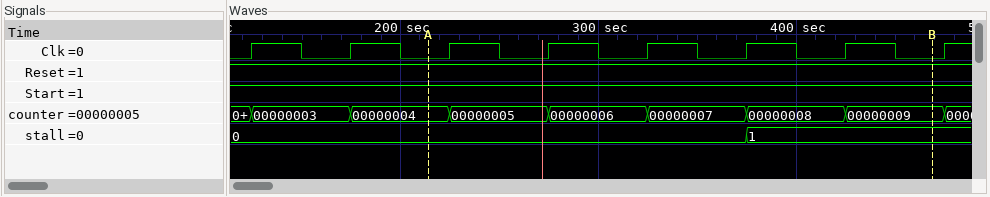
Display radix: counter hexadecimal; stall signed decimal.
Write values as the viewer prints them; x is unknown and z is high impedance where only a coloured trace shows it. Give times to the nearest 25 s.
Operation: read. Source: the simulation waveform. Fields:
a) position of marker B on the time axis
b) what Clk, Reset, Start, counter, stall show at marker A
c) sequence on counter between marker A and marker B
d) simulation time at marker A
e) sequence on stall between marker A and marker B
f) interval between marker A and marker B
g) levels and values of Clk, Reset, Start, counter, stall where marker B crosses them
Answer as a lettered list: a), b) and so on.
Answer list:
a) 475 s
b) Clk=0, Reset=1, Start=1, counter=00000004, stall=0
c) 00000004, 00000005, 00000006, 00000007, 00000008, 00000009
d) 225 s
e) 0, 1
f) 250 s
g) Clk=0, Reset=1, Start=1, counter=00000009, stall=1
